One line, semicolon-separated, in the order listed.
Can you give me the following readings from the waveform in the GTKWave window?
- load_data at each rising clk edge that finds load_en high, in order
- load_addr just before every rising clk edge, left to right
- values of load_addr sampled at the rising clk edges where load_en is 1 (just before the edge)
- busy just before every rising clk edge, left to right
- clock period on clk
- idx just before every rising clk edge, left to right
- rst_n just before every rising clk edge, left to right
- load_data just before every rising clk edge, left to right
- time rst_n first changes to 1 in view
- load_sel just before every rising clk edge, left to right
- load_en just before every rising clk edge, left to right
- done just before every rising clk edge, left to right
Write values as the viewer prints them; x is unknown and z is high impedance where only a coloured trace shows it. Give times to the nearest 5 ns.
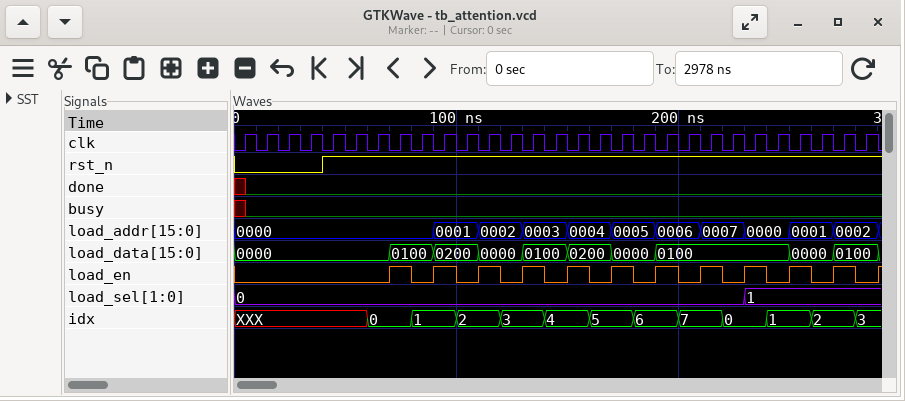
0100, 0200, 0000, 0100, 0200, 0000, 0100, 0100, 0100, 0000, 0100; 0000, 0000, 0000, 0000, 0000, 0000, 0000, 0000, 0000, 0001, 0001, 0002, 0002, 0003, 0003, 0004, 0004, 0005, 0005, 0006, 0006, 0007, 0007, 0000, 0000, 0001, 0001, 0002, 0002; 0000, 0001, 0002, 0003, 0004, 0005, 0006, 0007, 0000, 0001, 0002; x 0 0 0 0 0 0 0 0 0 0 0 0 0 0 0 0 0 0 0 0 0 0 0 0 0 0 0 0; 10 ns; XXX, XXX, XXX, XXX, XXX, XXX, 0, 0, 1, 1, 2, 2, 3, 3, 4, 4, 5, 5, 6, 6, 7, 7, 0, 0, 1, 1, 2, 2, 3; 0 0 0 0 1 1 1 1 1 1 1 1 1 1 1 1 1 1 1 1 1 1 1 1 1 1 1 1 1; 0000, 0000, 0000, 0000, 0000, 0000, 0000, 0100, 0100, 0200, 0200, 0000, 0000, 0100, 0100, 0200, 0200, 0000, 0000, 0100, 0100, 0100, 0100, 0100, 0100, 0000, 0000, 0100, 0100; 40 ns; 0, 0, 0, 0, 0, 0, 0, 0, 0, 0, 0, 0, 0, 0, 0, 0, 0, 0, 0, 0, 0, 0, 0, 1, 1, 1, 1, 1, 1; 0 0 0 0 0 0 0 1 0 1 0 1 0 1 0 1 0 1 0 1 0 1 0 1 0 1 0 1 0; x 0 0 0 0 0 0 0 0 0 0 0 0 0 0 0 0 0 0 0 0 0 0 0 0 0 0 0 0
